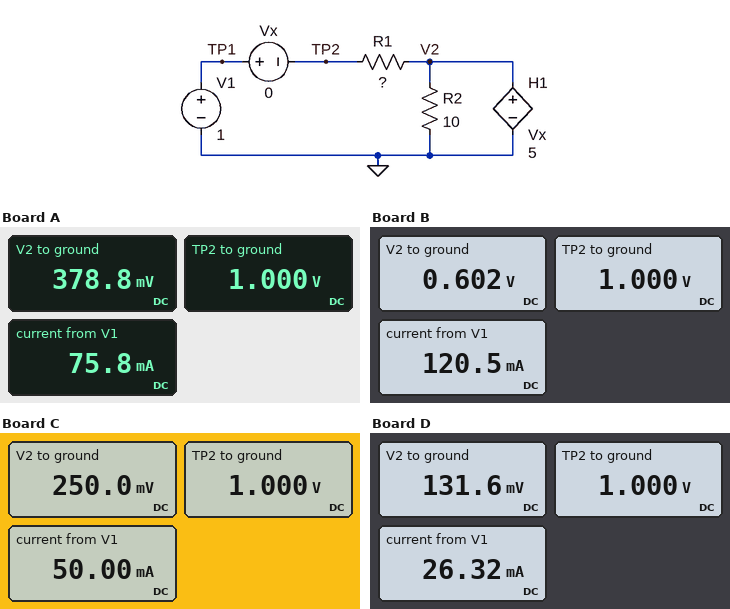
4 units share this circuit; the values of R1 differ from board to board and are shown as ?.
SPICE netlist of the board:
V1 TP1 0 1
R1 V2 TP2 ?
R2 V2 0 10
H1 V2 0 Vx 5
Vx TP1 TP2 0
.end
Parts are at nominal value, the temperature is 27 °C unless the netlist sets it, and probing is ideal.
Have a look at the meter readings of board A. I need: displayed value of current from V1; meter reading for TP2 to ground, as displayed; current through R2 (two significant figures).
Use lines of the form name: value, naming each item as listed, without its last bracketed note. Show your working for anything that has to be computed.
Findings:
displayed value of current from V1: 75.8 mA
meter reading for TP2 to ground, as displayed: 1.000 V
current through R2: (378.8 mV) / 10 Ω = 38 mA
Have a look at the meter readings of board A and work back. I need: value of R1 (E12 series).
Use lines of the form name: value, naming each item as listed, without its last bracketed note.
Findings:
value of R1: 8.2 Ω
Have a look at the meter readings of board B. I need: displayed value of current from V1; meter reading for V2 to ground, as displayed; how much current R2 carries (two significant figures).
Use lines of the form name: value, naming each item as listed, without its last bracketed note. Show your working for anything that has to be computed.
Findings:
displayed value of current from V1: 120.5 mA
meter reading for V2 to ground, as displayed: 0.602 V
how much current R2 carries: (602 mV) / 10 Ω = 60 mA
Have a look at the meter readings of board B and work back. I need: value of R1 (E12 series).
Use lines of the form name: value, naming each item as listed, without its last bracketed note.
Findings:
value of R1: 3.3 Ω
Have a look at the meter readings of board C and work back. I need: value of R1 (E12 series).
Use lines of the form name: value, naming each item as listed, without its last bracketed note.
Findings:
value of R1: 15 Ω
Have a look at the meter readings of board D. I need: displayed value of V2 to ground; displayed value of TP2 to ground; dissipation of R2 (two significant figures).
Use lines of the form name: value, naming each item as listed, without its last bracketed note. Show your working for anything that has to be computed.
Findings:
displayed value of V2 to ground: 131.6 mV
displayed value of TP2 to ground: 1.000 V
dissipation of R2: (131.6 mV)^2 / 10 Ω = 1.7 mW
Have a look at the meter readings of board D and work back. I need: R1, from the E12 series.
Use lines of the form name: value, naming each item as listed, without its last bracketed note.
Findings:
R1, from the E12 series: 33 Ω
